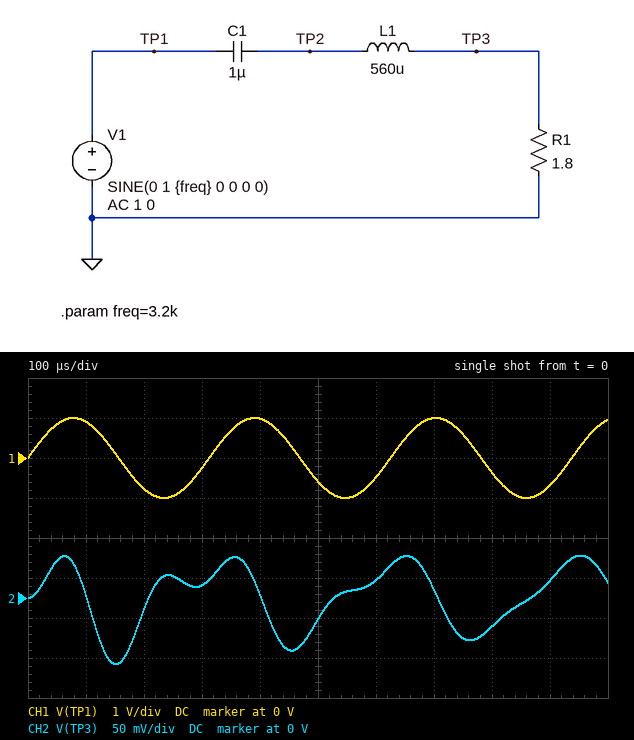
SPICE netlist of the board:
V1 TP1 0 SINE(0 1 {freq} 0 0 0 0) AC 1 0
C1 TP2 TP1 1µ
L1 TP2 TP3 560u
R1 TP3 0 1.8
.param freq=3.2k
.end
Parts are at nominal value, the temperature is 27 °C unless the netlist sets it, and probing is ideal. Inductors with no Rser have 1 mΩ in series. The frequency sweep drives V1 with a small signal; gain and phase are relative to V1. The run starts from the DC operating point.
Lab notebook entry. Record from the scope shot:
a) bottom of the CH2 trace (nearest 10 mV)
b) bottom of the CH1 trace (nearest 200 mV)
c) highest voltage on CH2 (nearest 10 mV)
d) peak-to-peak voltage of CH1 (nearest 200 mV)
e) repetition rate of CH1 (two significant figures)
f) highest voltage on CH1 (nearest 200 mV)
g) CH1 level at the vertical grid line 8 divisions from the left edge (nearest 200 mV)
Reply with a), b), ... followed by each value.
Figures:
a) -80 mV
b) -1.0 V
c) 50 mV
d) 2.0 V
e) 3.2 kHz
f) 1.0 V
g) -400 mV
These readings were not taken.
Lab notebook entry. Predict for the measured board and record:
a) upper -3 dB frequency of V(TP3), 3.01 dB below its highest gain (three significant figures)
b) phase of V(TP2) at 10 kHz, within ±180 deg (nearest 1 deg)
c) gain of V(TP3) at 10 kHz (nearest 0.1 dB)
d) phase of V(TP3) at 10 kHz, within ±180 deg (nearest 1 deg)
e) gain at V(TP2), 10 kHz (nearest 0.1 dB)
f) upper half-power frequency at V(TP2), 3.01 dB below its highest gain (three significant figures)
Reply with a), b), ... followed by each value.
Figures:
a) 6.99 kHz
b) 2 deg
c) -20.6 dB
d) -85 deg
e) 5.2 dB
f) 7.01 kHz
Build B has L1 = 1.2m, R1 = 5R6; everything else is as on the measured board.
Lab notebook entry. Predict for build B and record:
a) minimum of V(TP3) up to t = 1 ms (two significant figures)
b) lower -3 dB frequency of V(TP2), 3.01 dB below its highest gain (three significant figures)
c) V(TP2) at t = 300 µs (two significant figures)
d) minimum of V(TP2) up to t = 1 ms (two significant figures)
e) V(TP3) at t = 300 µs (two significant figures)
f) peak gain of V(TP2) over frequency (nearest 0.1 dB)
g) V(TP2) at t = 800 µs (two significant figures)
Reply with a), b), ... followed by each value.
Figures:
a) -270 mV
b) 4.29 kHz
c) 1.2 V
d) -1.4 V
e) 250 mV
f) 16.0 dB
g) -200 mV
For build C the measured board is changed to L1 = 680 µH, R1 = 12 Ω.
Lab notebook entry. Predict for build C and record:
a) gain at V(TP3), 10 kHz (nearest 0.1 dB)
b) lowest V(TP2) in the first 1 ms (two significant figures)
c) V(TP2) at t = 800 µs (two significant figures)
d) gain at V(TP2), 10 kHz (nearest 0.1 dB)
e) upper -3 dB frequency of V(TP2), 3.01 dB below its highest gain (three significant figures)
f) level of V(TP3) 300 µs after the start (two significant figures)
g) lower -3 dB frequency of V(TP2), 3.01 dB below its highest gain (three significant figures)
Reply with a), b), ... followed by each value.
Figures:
a) -7.8 dB
b) -680 mV
c) -300 mV
d) 3.6 dB
e) 8.80 kHz
f) 270 mV
g) 5.20 kHz
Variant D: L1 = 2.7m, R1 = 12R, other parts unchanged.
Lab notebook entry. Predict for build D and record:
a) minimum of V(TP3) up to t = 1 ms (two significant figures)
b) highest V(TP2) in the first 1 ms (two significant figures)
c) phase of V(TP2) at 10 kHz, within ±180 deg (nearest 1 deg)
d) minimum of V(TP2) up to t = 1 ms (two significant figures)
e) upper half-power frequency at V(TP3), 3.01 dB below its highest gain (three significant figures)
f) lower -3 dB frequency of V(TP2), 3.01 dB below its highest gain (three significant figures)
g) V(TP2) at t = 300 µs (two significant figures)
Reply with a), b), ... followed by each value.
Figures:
a) -850 mV
b) 4.0 V
c) 0 deg
d) -3.8 V
e) 3.44 kHz
f) 2.79 kHz
g) 1.8 V
